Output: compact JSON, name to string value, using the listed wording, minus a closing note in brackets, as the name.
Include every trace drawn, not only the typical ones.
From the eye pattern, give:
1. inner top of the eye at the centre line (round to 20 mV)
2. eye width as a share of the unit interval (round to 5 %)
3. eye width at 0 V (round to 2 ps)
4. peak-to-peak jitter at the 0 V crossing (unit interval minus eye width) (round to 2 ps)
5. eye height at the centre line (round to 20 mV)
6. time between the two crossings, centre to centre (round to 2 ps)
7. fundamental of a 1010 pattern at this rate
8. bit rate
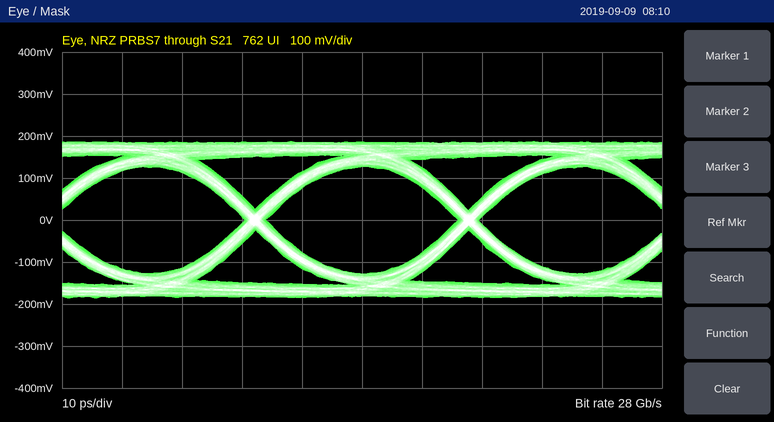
{"inner top of the eye at the centre line": "120 mV", "eye width as a share of the unit interval": "90 %", "eye width at 0 V": "32 ps", "peak-to-peak jitter at the 0 V crossing (unit interval minus eye width)": "4 ps", "eye height at the centre line": "260 mV", "time between the two crossings, centre to centre": "36 ps", "fundamental of a 1010 pattern at this rate": "14 GHz", "bit rate": "28 Gb/s"}
